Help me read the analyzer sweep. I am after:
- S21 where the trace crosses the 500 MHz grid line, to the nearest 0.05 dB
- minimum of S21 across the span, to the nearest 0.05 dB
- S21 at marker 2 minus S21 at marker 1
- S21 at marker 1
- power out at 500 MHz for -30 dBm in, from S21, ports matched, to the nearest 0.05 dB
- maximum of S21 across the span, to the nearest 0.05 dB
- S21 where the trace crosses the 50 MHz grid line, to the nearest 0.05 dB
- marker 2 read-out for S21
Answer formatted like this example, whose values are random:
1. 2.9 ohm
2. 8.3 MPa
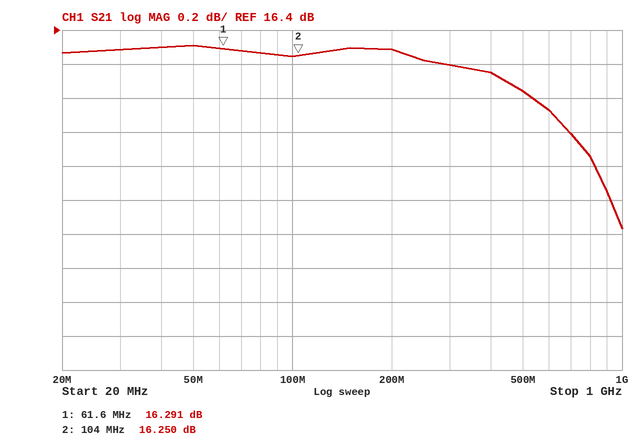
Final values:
1. 16.05 dB
2. 15.25 dB
3. -0.041 dB
4. 16.291 dB
5. -13.95 dBm
6. 16.30 dB
7. 16.30 dB
8. 16.250 dB
